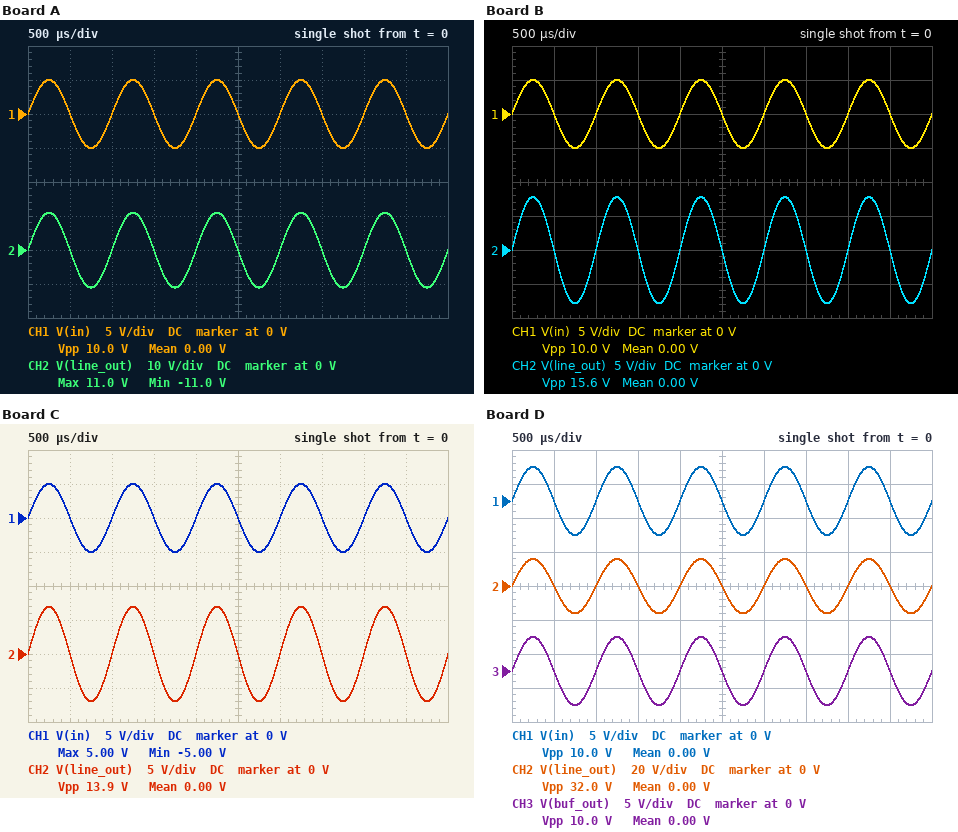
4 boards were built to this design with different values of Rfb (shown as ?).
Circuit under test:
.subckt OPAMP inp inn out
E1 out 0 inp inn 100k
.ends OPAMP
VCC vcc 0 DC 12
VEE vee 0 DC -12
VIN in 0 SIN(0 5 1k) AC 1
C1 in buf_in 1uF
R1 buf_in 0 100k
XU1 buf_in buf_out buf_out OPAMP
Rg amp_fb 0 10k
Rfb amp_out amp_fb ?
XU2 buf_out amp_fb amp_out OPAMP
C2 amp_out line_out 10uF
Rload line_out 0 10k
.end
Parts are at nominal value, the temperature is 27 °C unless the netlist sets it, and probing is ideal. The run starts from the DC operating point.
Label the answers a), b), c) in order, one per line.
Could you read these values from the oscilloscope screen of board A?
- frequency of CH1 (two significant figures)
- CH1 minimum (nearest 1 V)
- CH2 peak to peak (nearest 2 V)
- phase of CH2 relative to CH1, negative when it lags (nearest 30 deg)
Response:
a) 1.0 kHz
b) -5 V
c) 22 V
d) 0 deg
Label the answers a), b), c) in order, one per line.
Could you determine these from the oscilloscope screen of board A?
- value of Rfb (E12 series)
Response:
a) 12 kΩ
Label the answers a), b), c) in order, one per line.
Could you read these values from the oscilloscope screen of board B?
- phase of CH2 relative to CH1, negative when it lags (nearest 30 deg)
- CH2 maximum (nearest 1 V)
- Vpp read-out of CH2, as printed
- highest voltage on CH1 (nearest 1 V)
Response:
a) 0 deg
b) 8 V
c) 15.6 V
d) 5 V
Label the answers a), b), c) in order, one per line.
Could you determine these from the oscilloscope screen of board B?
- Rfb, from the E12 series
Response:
a) 5.6 kΩ
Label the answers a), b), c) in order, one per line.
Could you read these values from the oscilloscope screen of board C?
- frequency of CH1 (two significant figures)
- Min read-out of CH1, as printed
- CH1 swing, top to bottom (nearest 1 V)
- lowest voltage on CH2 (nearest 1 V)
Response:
a) 1.0 kHz
b) -5.00 V
c) 10 V
d) -7 V
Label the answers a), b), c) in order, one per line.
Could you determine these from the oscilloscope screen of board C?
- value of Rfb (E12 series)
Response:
a) 3.9 kΩ
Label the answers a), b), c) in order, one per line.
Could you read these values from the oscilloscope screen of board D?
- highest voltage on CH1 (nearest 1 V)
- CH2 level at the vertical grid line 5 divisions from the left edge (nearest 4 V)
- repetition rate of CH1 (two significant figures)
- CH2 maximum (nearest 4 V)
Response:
a) 5 V
b) 0 V
c) 1.0 kHz
d) 16 V
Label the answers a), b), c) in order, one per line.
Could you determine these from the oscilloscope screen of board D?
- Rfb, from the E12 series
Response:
a) 22 kΩ
